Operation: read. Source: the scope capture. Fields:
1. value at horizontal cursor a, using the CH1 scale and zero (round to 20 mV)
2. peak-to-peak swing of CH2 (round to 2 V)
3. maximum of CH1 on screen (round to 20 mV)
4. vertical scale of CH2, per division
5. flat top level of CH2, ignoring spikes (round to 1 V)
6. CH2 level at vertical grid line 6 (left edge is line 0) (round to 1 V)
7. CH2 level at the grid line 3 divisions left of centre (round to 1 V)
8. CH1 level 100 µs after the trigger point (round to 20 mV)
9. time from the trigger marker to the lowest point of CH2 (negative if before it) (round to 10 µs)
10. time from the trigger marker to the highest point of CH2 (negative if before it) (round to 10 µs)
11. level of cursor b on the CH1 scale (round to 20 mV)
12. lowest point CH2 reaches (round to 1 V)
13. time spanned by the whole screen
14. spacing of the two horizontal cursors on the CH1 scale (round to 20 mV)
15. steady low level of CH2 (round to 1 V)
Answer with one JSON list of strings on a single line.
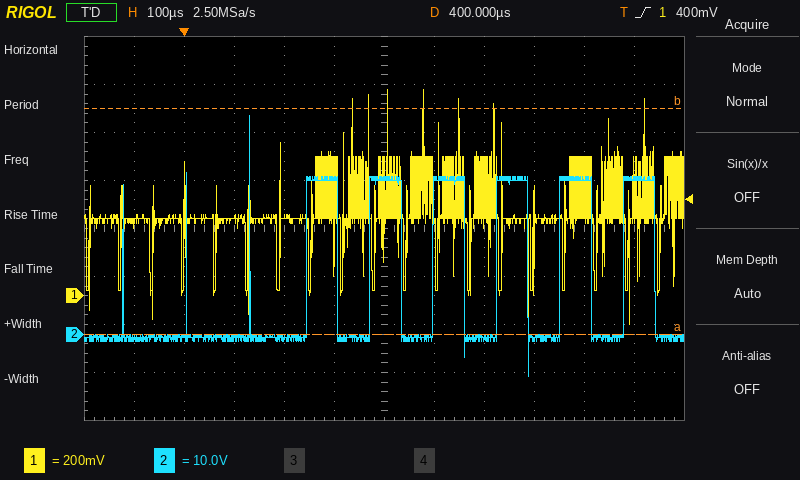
["-160 mV", "54 V", "860 mV", "10 V", "32 V", "32 V", "-1 V", "320 mV", "+690 µs", "+130 µs", "780 mV", "-9 V", "1.2 ms", "940 mV", "-1 V"]
